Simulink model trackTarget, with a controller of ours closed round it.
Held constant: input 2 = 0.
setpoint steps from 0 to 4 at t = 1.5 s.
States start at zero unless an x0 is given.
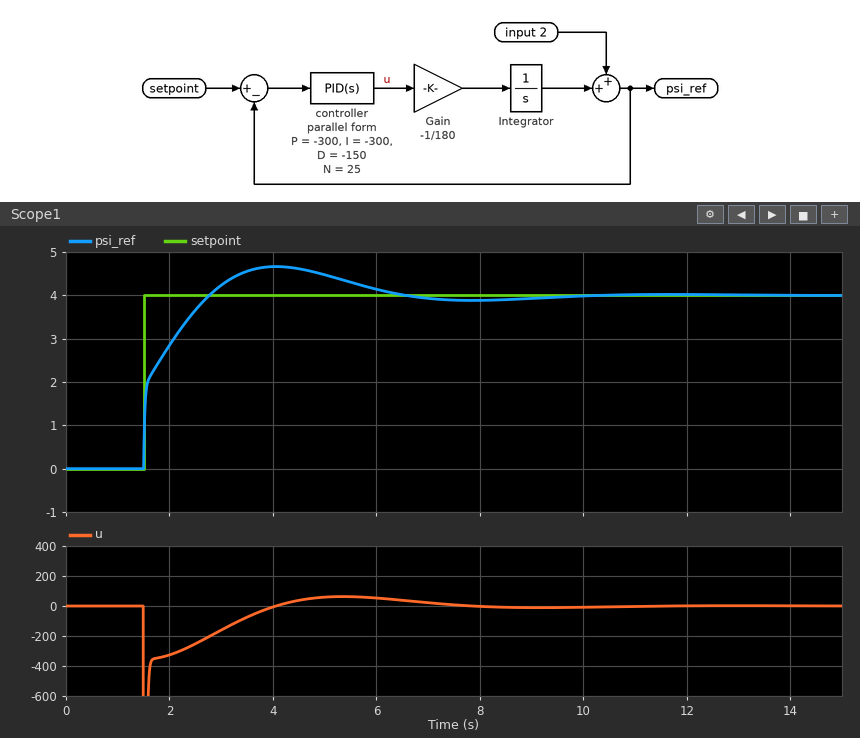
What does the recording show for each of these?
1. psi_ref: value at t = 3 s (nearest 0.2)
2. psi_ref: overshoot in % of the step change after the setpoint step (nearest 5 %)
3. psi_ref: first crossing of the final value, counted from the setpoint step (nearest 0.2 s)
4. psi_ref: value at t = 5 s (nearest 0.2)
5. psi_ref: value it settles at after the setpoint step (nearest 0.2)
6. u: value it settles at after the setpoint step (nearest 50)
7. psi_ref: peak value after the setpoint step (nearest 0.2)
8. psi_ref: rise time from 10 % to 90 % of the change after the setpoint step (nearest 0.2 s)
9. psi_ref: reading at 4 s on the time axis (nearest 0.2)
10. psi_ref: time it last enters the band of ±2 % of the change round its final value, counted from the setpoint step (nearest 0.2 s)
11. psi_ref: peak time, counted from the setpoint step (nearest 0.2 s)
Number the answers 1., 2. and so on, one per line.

1. 4.2
2. 15 %
3. 1.2 s
4. 4.4
5. 4.0
6. 0
7. 4.6
8. 1.0 s
9. 4.6
10. 7.4 s
11. 2.6 s
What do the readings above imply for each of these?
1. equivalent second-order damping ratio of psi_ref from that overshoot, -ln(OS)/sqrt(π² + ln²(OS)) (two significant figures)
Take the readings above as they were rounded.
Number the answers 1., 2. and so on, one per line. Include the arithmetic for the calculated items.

1. ln(0.15) = -1.897; 1.897 / sqrt(9.870 + 3.599) = 0.52
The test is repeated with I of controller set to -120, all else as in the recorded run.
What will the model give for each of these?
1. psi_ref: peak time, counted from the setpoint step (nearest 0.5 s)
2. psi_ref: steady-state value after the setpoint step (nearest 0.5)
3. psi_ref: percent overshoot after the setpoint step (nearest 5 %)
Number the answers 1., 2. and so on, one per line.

1. 3.5 s
2. 4.0
3. 10 %
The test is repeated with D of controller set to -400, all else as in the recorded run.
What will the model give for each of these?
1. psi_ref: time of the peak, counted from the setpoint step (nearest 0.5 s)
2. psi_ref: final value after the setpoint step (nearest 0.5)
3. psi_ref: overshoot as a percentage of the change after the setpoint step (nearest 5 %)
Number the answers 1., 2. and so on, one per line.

1. 3.5 s
2. 4.0
3. 10 %
